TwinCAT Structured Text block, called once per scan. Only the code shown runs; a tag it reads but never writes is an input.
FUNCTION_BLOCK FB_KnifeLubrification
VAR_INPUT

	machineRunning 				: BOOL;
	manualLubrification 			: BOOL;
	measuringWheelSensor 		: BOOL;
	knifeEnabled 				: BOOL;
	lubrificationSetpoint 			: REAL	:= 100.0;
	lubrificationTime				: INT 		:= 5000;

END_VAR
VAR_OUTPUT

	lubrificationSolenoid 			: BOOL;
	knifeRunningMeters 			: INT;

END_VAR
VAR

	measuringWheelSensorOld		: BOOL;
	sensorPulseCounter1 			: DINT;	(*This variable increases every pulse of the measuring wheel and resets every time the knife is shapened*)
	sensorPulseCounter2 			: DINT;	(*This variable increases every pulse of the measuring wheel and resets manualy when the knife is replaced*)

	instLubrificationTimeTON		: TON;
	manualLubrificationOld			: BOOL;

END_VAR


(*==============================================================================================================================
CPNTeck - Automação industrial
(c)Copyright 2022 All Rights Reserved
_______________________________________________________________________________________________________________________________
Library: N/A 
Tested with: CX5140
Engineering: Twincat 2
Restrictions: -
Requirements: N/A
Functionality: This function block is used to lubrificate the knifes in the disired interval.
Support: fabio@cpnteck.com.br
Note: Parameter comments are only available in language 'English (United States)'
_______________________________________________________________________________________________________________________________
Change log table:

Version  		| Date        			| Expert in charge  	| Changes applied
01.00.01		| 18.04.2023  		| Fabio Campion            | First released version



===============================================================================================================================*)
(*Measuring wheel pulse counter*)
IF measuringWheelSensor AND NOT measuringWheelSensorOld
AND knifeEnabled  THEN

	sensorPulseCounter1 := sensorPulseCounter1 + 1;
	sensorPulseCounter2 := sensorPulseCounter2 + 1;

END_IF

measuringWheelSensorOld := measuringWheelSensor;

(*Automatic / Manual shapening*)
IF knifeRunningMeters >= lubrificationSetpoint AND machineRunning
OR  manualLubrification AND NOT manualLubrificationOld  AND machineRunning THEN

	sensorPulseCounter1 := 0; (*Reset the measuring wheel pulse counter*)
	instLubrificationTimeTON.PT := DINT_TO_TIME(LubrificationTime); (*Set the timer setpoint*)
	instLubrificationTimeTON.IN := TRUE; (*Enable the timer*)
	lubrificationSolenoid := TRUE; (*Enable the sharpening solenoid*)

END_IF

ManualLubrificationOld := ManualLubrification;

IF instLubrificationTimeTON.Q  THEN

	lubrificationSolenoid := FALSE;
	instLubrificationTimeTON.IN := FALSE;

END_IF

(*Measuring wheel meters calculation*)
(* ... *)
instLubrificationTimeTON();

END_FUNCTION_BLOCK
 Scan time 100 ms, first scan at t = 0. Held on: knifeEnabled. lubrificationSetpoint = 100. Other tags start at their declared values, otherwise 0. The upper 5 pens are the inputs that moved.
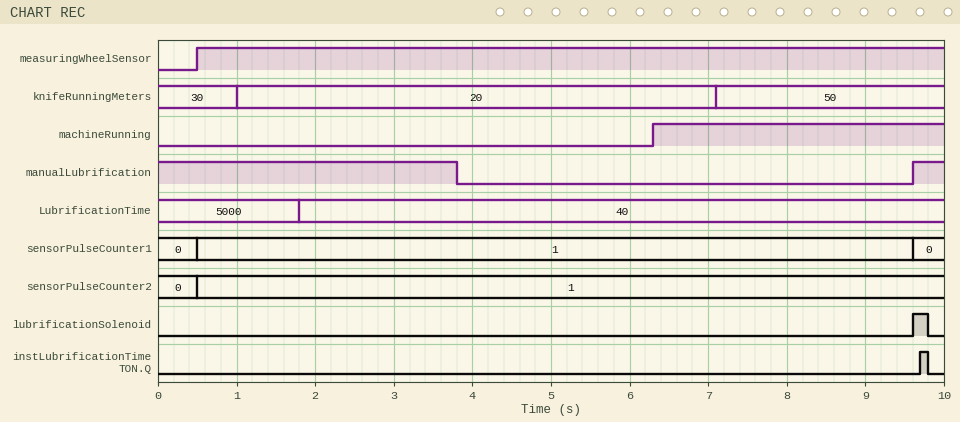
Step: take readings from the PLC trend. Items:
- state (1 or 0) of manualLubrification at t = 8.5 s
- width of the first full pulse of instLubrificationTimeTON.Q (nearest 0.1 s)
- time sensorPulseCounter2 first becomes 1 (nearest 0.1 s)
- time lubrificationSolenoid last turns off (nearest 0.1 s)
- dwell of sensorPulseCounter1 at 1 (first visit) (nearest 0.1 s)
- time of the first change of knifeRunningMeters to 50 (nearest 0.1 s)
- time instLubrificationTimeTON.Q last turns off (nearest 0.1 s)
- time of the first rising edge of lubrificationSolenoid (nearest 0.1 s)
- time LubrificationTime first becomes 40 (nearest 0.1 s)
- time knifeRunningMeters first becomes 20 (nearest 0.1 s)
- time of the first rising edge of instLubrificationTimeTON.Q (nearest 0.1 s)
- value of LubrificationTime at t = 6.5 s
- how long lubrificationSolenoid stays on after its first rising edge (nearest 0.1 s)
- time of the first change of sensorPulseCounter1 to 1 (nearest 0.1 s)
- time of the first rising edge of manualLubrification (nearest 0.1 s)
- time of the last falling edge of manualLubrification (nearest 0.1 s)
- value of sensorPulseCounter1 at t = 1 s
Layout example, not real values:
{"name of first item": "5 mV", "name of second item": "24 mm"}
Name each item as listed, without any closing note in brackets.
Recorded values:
{"state (1 or 0) of manualLubrification at t = 8.5 s": "0", "width of the first full pulse of instLubrificationTimeTON.Q": "0.1 s", "time sensorPulseCounter2 first becomes 1": "0.5 s", "time lubrificationSolenoid last turns off": "9.8 s", "dwell of sensorPulseCounter1 at 1 (first visit)": "9.1 s", "time of the first change of knifeRunningMeters to 50": "7.1 s", "time instLubrificationTimeTON.Q last turns off": "9.8 s", "time of the first rising edge of lubrificationSolenoid": "9.6 s", "time LubrificationTime first becomes 40": "1.8 s", "time knifeRunningMeters first becomes 20": "1.0 s", "time of the first rising edge of instLubrificationTimeTON.Q": "9.7 s", "value of LubrificationTime at t = 6.5 s": "40", "how long lubrificationSolenoid stays on after its first rising edge": "0.2 s", "time of the first change of sensorPulseCounter1 to 1": "0.5 s", "time of the first rising edge of manualLubrification": "9.6 s", "time of the last falling edge of manualLubrification": "3.8 s", "value of sensorPulseCounter1 at t = 1 s": "1"}
